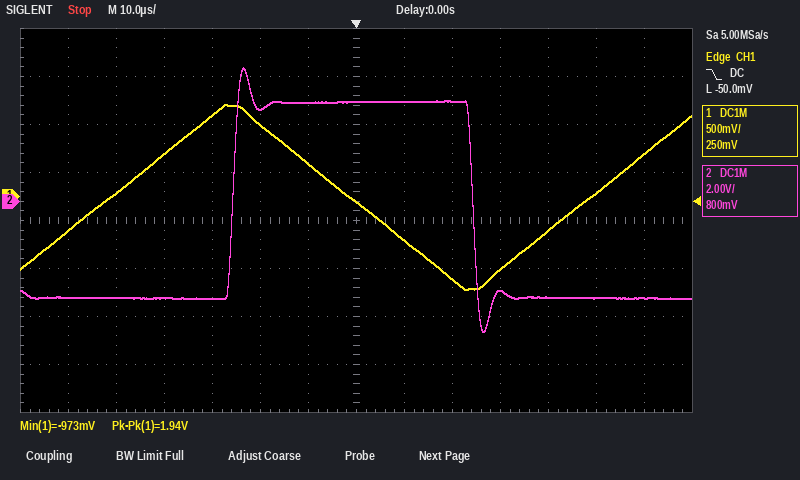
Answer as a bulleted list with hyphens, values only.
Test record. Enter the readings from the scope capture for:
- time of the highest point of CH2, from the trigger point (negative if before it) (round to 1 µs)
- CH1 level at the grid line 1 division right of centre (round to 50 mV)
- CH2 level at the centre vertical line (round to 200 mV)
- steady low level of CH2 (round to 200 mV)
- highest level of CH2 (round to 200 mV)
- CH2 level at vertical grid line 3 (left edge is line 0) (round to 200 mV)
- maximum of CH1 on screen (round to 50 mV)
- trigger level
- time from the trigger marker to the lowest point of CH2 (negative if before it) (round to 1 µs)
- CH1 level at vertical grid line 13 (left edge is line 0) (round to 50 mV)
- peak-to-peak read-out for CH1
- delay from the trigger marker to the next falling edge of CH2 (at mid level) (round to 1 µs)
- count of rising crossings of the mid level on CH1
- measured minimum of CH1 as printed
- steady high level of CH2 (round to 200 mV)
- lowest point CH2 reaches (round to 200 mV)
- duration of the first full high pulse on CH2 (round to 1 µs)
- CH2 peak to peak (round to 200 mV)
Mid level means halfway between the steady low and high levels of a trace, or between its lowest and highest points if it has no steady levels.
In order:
- -23 µs
- -450 mV
- 4.2 V
- -4.0 V
- 5.6 V
- -4.0 V
- 950 mV
- -50.0 mV
- +27 µs
- 450 mV
- 1.94 V
- 24 µs
- 2
- -973 mV
- 4.2 V
- -5.4 V
- 50 µs
- 11.0 V
